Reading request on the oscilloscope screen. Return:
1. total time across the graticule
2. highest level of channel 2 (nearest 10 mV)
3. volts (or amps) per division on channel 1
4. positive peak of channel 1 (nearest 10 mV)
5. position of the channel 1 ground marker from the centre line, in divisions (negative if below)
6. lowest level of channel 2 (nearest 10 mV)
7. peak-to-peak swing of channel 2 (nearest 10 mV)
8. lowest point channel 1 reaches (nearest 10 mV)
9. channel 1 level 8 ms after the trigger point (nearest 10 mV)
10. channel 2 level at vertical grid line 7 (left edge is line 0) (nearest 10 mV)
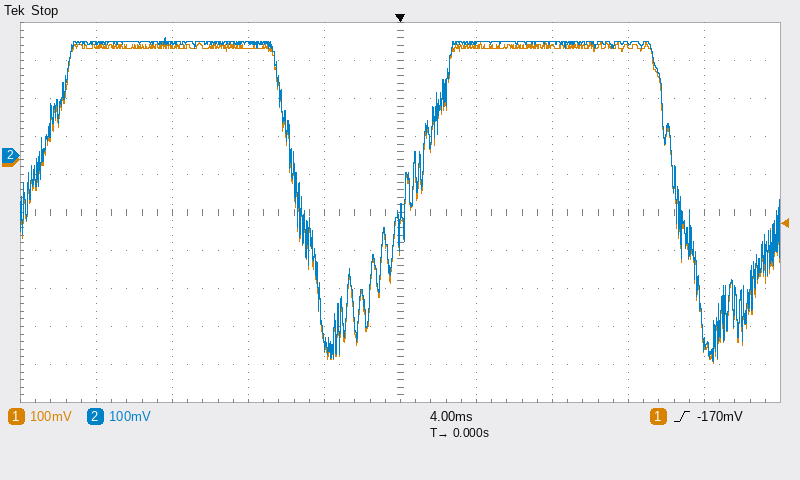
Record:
40 ms
310 mV
100 mV
310 mV
+1.4 div
-540 mV
850 mV
-540 mV
300 mV
300 mV
